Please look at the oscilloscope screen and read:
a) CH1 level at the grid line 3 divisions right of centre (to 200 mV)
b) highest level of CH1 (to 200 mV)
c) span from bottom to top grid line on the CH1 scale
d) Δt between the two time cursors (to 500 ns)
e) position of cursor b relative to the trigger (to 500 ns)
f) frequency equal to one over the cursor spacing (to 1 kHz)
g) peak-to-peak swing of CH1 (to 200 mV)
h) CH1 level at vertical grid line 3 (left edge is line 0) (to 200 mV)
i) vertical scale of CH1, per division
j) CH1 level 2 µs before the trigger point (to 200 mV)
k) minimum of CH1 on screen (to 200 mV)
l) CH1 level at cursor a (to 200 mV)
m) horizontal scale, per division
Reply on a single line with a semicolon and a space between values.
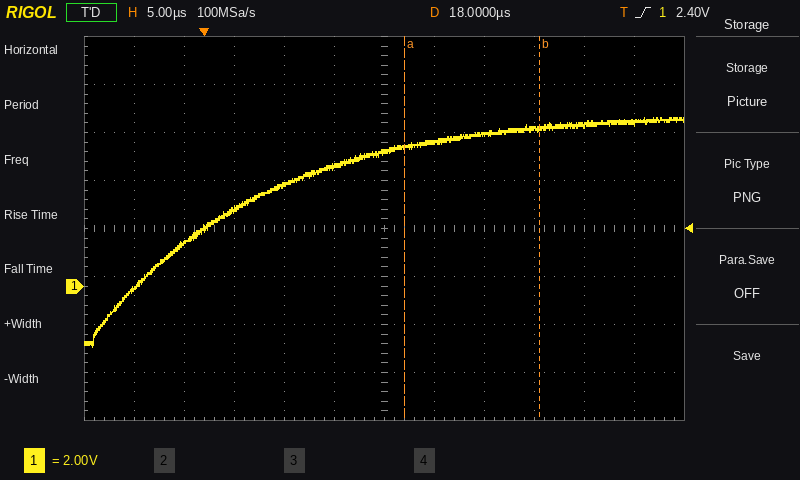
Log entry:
6.6 V; 7.0 V; 16 V; 13.5 µs; +33.5 µs; 74 kHz; 9.6 V; 3.2 V; 2 V; 1.8 V; -2.6 V; 5.8 V; 5 µs
